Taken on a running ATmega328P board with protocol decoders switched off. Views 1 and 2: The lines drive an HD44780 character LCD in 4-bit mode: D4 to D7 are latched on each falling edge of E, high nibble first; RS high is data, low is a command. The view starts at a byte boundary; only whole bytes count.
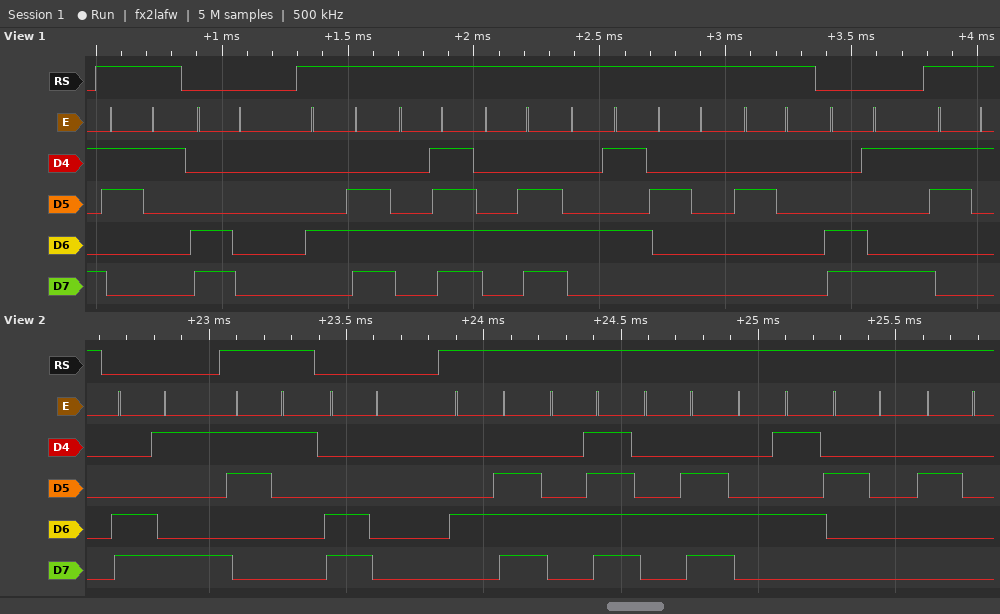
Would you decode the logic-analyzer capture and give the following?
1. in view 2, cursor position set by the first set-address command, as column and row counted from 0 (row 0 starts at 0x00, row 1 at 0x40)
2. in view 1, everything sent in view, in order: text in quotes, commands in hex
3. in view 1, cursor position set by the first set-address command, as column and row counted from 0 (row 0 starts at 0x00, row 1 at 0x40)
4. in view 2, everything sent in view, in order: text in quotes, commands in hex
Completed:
column 9, row 1
"1" 0xC0 "NONE  " 0xC9 "1"
column 0, row 1
0xC9 "1" 0xC0 "NONE  "
